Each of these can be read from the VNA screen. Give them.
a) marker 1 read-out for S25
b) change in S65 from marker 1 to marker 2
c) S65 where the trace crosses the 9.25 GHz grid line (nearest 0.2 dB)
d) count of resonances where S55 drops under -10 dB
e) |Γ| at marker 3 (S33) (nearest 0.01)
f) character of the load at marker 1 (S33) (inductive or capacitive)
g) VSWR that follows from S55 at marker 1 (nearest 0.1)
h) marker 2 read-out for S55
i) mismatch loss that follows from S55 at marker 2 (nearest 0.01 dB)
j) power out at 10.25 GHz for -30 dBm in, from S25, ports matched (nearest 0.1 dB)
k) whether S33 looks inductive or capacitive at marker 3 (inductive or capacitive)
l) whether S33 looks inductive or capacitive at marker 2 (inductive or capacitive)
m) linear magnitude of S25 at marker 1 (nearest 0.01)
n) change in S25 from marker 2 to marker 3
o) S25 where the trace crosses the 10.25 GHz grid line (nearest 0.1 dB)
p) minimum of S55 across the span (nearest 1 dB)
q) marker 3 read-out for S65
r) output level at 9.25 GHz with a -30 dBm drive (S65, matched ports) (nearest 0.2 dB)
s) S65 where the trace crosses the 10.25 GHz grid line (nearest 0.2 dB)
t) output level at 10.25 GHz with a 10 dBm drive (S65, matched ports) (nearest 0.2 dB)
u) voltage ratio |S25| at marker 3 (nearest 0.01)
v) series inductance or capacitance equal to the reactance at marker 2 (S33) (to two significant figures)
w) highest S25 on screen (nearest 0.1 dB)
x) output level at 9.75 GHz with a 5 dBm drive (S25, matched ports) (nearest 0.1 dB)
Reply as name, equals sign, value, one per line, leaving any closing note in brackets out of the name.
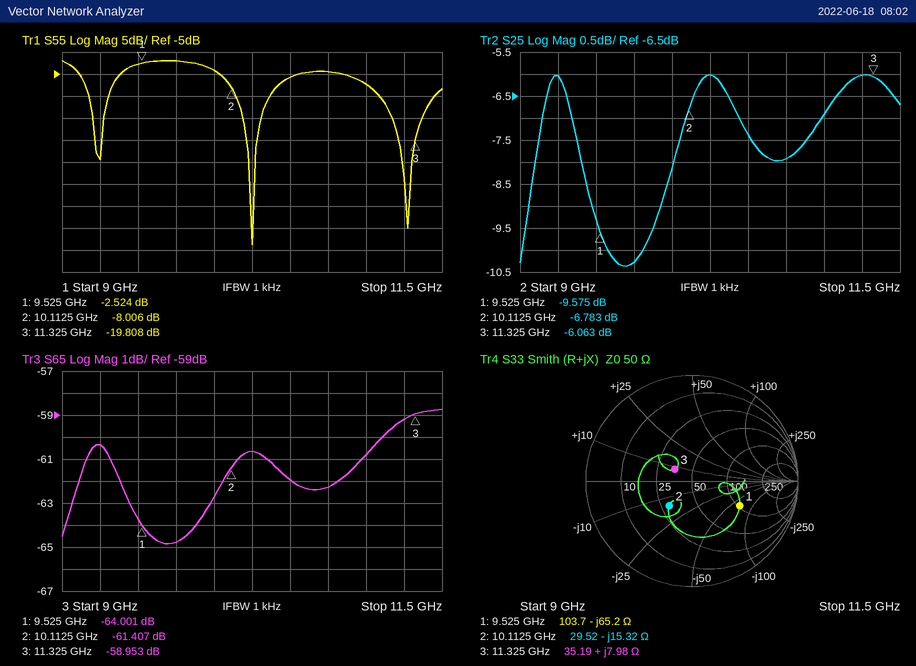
marker 1 read-out for S25 = -9.575 dB
change in S65 from marker 1 to marker 2 = 2.594 dB
S65 where the trace crosses the 9.25 GHz grid line = -60.4 dB
count of resonances where S55 drops under -10 dB = 3
|Γ| at marker 3 (S33) = 0.20
character of the load at marker 1 (S33) = capacitive
VSWR that follows from S55 at marker 1 = 6.9
marker 2 read-out for S55 = -8.006 dB
mismatch loss that follows from S55 at marker 2 = 0.75 dB
power out at 10.25 GHz for -30 dBm in, from S25, ports matched = -36.0 dBm
whether S33 looks inductive or capacitive at marker 3 = inductive
whether S33 looks inductive or capacitive at marker 2 = capacitive
linear magnitude of S25 at marker 1 = 0.33
change in S25 from marker 2 to marker 3 = 0.720 dB
S25 where the trace crosses the 10.25 GHz grid line = -6.0 dB
minimum of S55 across the span = -44 dB
marker 3 read-out for S65 = -58.953 dB
output level at 9.25 GHz with a -30 dBm drive (S65, matched ports) = -90.4 dBm
S65 where the trace crosses the 10.25 GHz grid line = -60.6 dB
output level at 10.25 GHz with a 10 dBm drive (S65, matched ports) = -50.6 dBm
voltage ratio |S25| at marker 3 = 0.50
series inductance or capacitance equal to the reactance at marker 2 (S33) = 1.0 pF
highest S25 on screen = -6.0 dB
output level at 9.75 GHz with a 5 dBm drive (S25, matched ports) = -5.3 dBm
